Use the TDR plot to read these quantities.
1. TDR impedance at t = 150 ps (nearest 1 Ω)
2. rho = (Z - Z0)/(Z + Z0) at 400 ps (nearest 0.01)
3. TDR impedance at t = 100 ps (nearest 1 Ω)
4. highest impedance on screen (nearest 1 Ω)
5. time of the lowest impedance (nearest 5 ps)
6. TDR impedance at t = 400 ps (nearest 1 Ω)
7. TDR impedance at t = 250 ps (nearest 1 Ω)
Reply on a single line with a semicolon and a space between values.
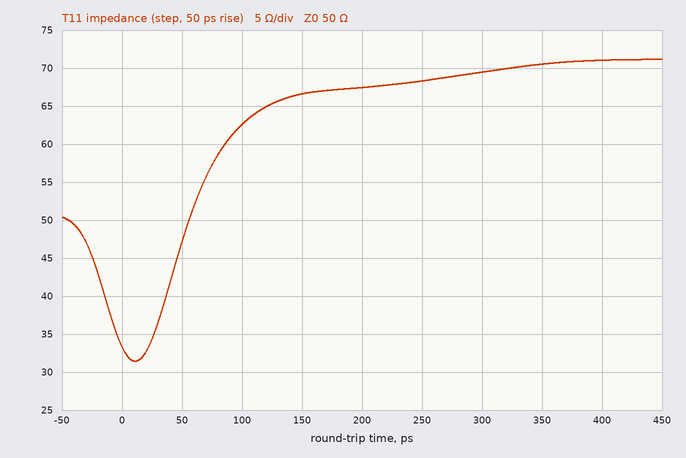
67 Ω; +0.17; 63 Ω; 71 Ω; 10 ps; 71 Ω; 68 Ω
